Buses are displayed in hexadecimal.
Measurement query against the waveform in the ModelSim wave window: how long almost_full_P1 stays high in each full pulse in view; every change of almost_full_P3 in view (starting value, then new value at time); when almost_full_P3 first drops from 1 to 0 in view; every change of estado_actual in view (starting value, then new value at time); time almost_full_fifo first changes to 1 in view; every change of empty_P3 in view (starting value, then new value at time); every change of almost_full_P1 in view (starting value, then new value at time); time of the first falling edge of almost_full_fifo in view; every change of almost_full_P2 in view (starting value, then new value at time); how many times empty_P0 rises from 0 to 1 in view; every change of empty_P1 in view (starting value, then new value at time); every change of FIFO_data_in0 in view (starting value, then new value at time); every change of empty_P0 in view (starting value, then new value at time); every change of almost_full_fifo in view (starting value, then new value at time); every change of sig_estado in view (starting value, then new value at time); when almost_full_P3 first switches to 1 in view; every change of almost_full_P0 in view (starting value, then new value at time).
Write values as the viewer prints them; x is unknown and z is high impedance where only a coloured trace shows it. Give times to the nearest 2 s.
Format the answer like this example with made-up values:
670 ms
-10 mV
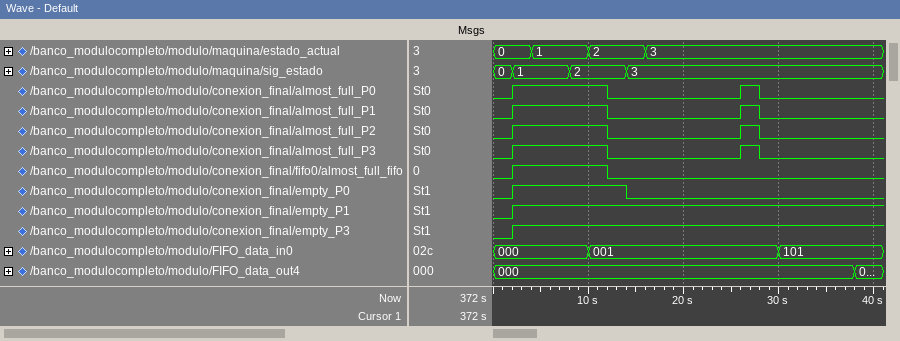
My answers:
10 s, 2 s
0, 1 at 2 s, 0 at 12 s, 1 at 26 s, 0 at 28 s
12 s
0, 1 at 4 s, 2 at 10 s, 3 at 16 s
2 s
0, 1 at 2 s
0, 1 at 2 s, 0 at 12 s, 1 at 26 s, 0 at 28 s
12 s
0, 1 at 2 s, 0 at 12 s, 1 at 26 s, 0 at 28 s
1
0, 1 at 2 s
000, 001 at 10 s, 101 at 30 s
0, 1 at 2 s, 0 at 14 s
0, 1 at 2 s, 0 at 12 s
0, 1 at 2 s, 2 at 8 s, 3 at 14 s
2 s
0, 1 at 2 s, 0 at 12 s, 1 at 26 s, 0 at 28 s
